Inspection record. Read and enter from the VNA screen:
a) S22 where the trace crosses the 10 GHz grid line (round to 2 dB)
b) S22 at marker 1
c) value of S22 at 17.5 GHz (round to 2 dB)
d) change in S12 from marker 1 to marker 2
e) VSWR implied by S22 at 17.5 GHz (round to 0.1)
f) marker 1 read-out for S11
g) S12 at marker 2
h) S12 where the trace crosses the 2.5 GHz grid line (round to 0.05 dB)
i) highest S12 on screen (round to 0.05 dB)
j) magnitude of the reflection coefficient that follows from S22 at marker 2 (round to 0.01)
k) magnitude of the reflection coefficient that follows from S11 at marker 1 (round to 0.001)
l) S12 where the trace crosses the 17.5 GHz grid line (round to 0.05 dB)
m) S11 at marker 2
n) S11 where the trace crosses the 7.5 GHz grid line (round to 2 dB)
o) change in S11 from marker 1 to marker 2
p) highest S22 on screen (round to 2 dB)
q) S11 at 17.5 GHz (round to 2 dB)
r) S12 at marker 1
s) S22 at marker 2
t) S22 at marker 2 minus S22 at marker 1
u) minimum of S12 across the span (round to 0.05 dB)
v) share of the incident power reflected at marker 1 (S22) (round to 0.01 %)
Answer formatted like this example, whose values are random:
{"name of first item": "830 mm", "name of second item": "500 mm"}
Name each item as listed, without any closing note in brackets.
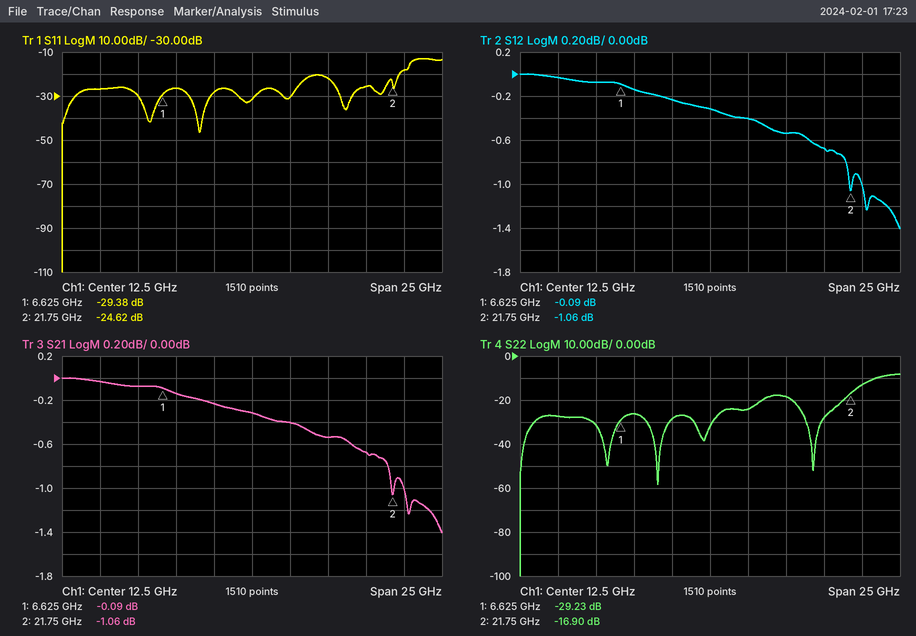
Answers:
{"S22 where the trace crosses the 10 GHz grid line": "-28 dB", "S22 at marker 1": "-29.23 dB", "value of S22 at 17.5 GHz": "-18 dB", "change in S12 from marker 1 to marker 2": "-0.97 dB", "VSWR implied by S22 at 17.5 GHz": "1.3", "marker 1 read-out for S11": "-29.38 dB", "S12 at marker 2": "-1.06 dB", "S12 where the trace crosses the 2.5 GHz grid line": "-0.05 dB", "highest S12 on screen": "0.00 dB", "magnitude of the reflection coefficient that follows from S22 at marker 2": "0.14", "magnitude of the reflection coefficient that follows from S11 at marker 1": "0.034", "S12 where the trace crosses the 17.5 GHz grid line": "-0.55 dB", "S11 at marker 2": "-24.62 dB", "S11 where the trace crosses the 7.5 GHz grid line": "-26 dB", "change in S11 from marker 1 to marker 2": "4.76 dB", "highest S22 on screen": "-8 dB", "S11 at 17.5 GHz": "-22 dB", "S12 at marker 1": "-0.09 dB", "S22 at marker 2": "-16.90 dB", "S22 at marker 2 minus S22 at marker 1": "12.33 dB", "minimum of S12 across the span": "-1.40 dB", "share of the incident power reflected at marker 1 (S22)": "0.12 %"}
